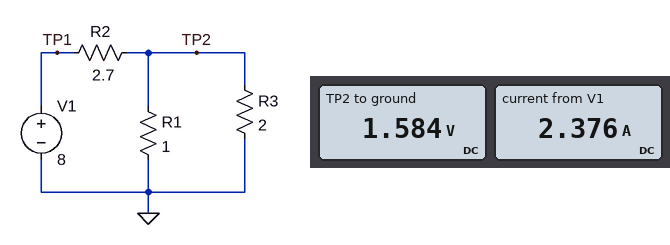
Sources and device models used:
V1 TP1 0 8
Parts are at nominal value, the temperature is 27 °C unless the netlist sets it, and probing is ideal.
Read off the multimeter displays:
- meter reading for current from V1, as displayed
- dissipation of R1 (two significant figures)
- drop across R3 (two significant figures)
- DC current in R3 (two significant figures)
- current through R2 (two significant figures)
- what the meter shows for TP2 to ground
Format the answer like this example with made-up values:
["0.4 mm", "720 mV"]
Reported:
["2.376 A", "2.5 W", "1.6 V", "790 mA", "2.4 A", "1.584 V"]
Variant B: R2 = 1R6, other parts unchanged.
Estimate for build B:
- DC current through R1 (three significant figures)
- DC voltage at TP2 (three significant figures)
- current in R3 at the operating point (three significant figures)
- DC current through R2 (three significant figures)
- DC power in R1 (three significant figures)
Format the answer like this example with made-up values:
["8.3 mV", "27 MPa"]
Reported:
["2.35 A", "2.35 V", "1.18 A", "3.53 A", "5.54 W"]
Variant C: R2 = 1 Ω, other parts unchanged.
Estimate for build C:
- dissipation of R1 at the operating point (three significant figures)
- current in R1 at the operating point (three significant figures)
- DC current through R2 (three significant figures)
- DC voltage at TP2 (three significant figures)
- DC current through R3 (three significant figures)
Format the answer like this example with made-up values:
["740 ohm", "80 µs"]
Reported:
["10.2 W", "3.20 A", "4.80 A", "3.20 V", "1.60 A"]
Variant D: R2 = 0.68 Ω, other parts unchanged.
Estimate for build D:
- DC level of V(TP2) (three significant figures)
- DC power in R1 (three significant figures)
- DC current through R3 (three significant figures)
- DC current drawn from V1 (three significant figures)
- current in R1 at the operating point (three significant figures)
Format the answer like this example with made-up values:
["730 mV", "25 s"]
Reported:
["3.96 V", "15.7 W", "1.98 A", "5.94 A", "3.96 A"]
